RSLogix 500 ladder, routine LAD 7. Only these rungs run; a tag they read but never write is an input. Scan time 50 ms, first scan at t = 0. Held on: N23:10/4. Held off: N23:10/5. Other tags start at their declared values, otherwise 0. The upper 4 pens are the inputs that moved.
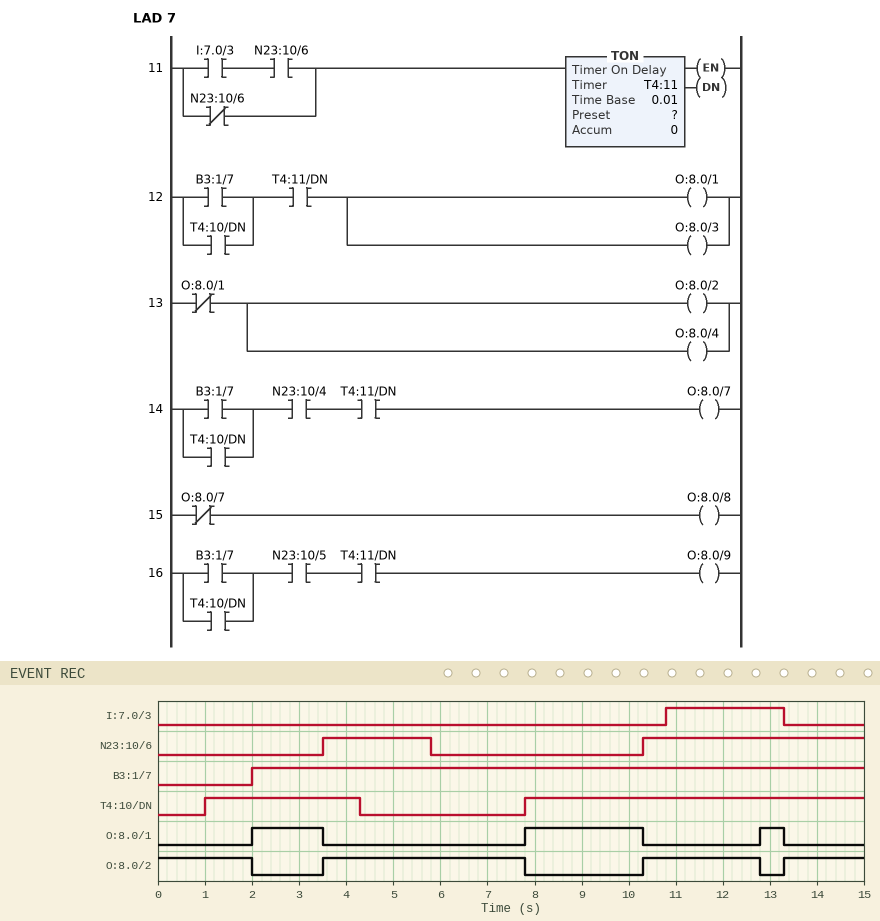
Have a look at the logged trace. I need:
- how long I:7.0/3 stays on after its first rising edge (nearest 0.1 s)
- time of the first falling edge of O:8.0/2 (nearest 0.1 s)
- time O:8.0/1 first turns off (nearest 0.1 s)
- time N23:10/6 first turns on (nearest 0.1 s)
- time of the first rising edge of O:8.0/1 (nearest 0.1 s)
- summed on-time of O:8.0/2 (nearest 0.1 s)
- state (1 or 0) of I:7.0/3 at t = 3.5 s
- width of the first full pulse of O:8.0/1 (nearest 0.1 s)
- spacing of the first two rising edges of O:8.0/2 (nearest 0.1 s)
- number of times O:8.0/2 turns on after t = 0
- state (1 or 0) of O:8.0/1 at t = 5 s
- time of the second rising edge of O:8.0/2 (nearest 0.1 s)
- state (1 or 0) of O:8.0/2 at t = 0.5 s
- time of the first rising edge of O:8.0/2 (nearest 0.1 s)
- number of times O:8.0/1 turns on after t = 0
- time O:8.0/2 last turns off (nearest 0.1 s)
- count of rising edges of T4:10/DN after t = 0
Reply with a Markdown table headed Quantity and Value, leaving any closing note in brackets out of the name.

| Quantity | Value |
|---|---|
| how long I:7.0/3 stays on after its first rising edge | 2.5 s |
| time of the first falling edge of O:8.0/2 | 2.0 s |
| time O:8.0/1 first turns off | 3.5 s |
| time N23:10/6 first turns on | 3.5 s |
| time of the first rising edge of O:8.0/1 | 2.0 s |
| summed on-time of O:8.0/2 | 10.5 s |
| state (1 or 0) of I:7.0/3 at t = 3.5 s | 0 |
| width of the first full pulse of O:8.0/1 | 1.5 s |
| spacing of the first two rising edges of O:8.0/2 | 6.8 s |
| number of times O:8.0/2 turns on after t = 0 | 3 |
| state (1 or 0) of O:8.0/1 at t = 5 s | 0 |
| time of the second rising edge of O:8.0/2 | 10.3 s |
| state (1 or 0) of O:8.0/2 at t = 0.5 s | 1 |
| time of the first rising edge of O:8.0/2 | 3.5 s |
| number of times O:8.0/1 turns on after t = 0 | 3 |
| time O:8.0/2 last turns off | 12.8 s |
| count of rising edges of T4:10/DN after t = 0 | 2 |
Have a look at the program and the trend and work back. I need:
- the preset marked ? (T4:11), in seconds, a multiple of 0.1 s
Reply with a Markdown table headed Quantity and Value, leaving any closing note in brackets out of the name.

| Quantity | Value |
|---|---|
| the preset marked ? (T4:11), in seconds, a multiple of 0.1 s | 2.0 s |
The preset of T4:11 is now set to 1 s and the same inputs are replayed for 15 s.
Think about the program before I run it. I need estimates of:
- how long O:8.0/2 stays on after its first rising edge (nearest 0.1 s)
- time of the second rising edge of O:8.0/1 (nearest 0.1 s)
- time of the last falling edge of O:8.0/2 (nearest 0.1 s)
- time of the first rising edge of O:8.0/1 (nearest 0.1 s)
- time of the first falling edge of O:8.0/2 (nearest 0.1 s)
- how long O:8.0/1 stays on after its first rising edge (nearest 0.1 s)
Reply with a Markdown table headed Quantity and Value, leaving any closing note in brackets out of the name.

| Quantity | Value |
|---|---|
| how long O:8.0/2 stays on after its first rising edge | 3.3 s |
| time of the second rising edge of O:8.0/1 | 6.8 s |
| time of the last falling edge of O:8.0/2 | 11.8 s |
| time of the first rising edge of O:8.0/1 | 1.0 s |
| time of the first falling edge of O:8.0/2 | 1.0 s |
| how long O:8.0/1 stays on after its first rising edge | 2.5 s |
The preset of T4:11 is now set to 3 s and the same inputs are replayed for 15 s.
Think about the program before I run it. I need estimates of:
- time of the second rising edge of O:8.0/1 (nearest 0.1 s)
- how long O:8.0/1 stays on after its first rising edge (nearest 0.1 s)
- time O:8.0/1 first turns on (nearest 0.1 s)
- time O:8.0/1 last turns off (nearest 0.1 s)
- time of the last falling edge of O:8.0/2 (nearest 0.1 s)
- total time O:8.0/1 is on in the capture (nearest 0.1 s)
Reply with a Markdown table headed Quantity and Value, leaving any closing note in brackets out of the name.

| Quantity | Value |
|---|---|
| time of the second rising edge of O:8.0/1 | 8.8 s |
| how long O:8.0/1 stays on after its first rising edge | 0.5 s |
| time O:8.0/1 first turns on | 3.0 s |
| time O:8.0/1 last turns off | 10.3 s |
| time of the last falling edge of O:8.0/2 | 8.8 s |
| total time O:8.0/1 is on in the capture | 2.0 s |
